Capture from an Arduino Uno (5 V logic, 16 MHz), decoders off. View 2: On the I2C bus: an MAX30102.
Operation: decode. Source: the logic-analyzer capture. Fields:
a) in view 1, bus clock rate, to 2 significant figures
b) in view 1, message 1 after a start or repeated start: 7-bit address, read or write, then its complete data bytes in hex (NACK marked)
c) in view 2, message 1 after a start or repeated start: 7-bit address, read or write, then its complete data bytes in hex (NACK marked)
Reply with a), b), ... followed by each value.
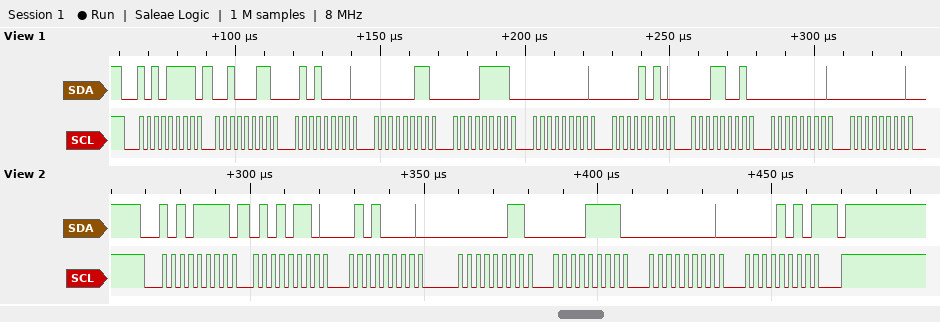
a) 400 kHz
b) 0x57 read: 23 50 03 0F 00 0A 19 00 00
c) 0x57 read: 56 50 03 0F 00 0A NACK
